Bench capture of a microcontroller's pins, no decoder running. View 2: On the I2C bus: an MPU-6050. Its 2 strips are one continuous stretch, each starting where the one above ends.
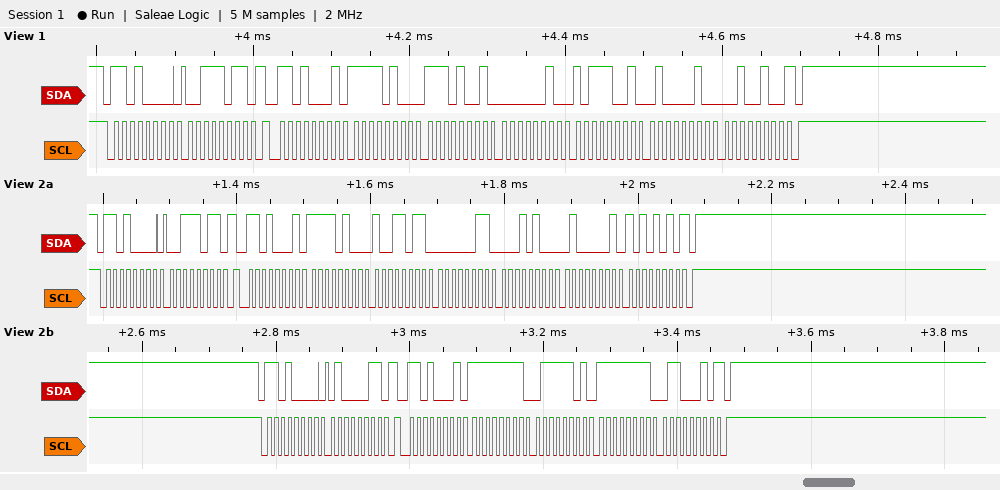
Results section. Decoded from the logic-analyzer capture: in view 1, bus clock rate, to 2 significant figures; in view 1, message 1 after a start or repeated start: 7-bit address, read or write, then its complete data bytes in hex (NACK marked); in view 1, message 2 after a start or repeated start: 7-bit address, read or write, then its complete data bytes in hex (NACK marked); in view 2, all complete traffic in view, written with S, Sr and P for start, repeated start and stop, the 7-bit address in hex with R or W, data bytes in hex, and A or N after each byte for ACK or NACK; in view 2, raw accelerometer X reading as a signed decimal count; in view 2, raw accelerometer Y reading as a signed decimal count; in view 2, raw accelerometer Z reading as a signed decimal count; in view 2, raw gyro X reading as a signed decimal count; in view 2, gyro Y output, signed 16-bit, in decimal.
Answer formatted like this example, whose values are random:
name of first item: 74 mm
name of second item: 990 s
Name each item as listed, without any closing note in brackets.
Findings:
in view 1, bus clock rate, to 2 significant figures: 100 kHz
in view 1, message 1 after a start or repeated start: 7-bit address, read or write, then its complete data bytes in hex: 0x68 write: 3B
in view 1, message 2 after a start or repeated start: 7-bit address, read or write, then its complete data bytes in hex: 0x68 read: F4 E9 02 B9 42 24 NACK
in view 2, all complete traffic in view, written with S, Sr and P for start, repeated start and stop, the 7-bit address in hex with R or W, data bytes in hex, and A or N after each byte for ACK or NACK: S 68W A 3B A Sr 68R A F4 A 9B A 03 A 14 A 41 A AA N P S 68W A 43 A Sr 68R A FF A 7D A FF A 62 N P
in view 2, raw accelerometer X reading as a signed decimal count: -2917
in view 2, raw accelerometer Y reading as a signed decimal count: 788
in view 2, raw accelerometer Z reading as a signed decimal count: 16810
in view 2, raw gyro X reading as a signed decimal count: -131
in view 2, gyro Y output, signed 16-bit, in decimal: -158
